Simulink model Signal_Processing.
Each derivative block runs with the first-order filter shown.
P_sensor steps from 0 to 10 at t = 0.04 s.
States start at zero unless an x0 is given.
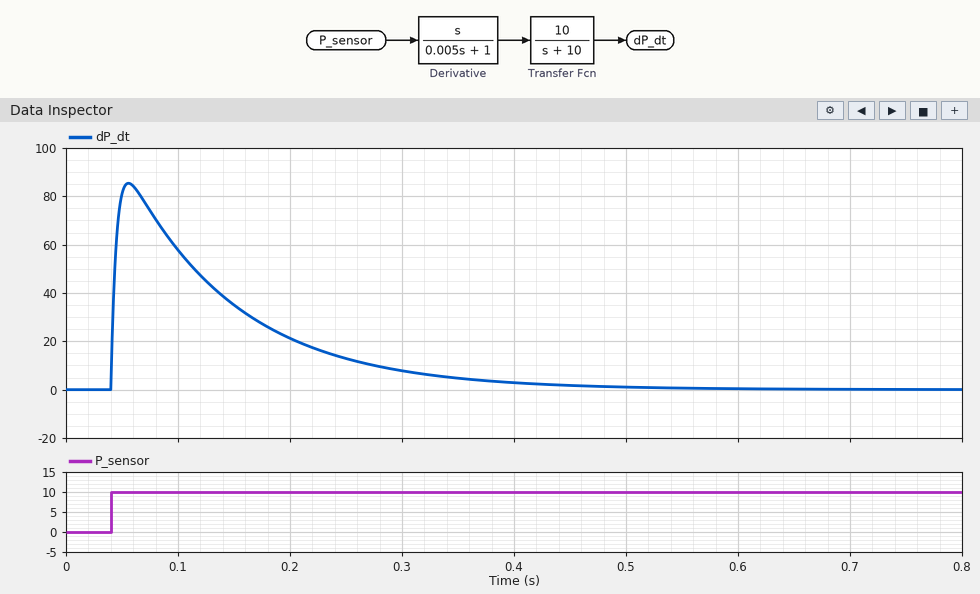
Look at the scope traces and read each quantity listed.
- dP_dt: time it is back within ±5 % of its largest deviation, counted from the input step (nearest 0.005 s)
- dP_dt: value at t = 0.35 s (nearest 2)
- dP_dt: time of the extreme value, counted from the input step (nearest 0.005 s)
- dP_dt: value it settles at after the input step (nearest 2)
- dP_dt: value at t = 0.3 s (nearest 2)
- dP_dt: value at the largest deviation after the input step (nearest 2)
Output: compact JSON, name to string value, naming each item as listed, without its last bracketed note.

{"dP_dt: time it is back within ±5 % of its largest deviation, counted from the input step": "0.320 s", "dP_dt: value at t = 0.35 s": "4", "dP_dt: time of the extreme value, counted from the input step": "0.015 s", "dP_dt: value it settles at after the input step": "0", "dP_dt: value at t = 0.3 s": "8", "dP_dt: value at the largest deviation after the input step": "86"}
